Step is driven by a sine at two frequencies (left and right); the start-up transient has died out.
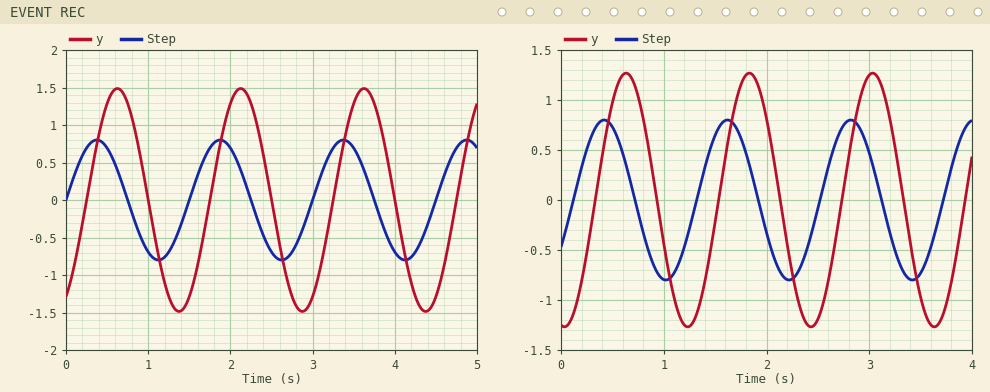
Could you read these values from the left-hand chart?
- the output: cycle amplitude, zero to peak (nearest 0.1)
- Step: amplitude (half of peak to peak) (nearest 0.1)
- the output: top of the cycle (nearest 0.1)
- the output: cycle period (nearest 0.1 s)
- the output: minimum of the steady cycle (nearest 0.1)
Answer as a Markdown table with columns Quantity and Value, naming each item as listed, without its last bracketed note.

| Quantity | Value |
|---|---|
| the output: cycle amplitude, zero to peak | 1.5 |
| Step: amplitude (half of peak to peak) | 0.8 |
| the output: top of the cycle | 1.5 |
| the output: cycle period | 1.5 s |
| the output: minimum of the steady cycle | -1.5 |
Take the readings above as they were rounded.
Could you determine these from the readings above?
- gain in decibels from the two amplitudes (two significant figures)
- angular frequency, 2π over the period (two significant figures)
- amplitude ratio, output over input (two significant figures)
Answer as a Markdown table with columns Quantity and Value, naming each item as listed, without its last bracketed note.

| Quantity | Value |
|---|---|
| gain in decibels from the two amplitudes | 5.5 dB |
| angular frequency, 2π over the period | 4.2 rad/s |
| amplitude ratio, output over input | 1.9 |
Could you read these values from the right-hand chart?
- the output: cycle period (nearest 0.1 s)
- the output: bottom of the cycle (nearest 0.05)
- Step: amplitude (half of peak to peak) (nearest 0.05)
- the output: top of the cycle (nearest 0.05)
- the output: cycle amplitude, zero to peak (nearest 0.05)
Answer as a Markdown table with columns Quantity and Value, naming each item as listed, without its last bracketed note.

| Quantity | Value |
|---|---|
| the output: cycle period | 1.2 s |
| the output: bottom of the cycle | -1.25 |
| Step: amplitude (half of peak to peak) | 0.80 |
| the output: top of the cycle | 1.25 |
| the output: cycle amplitude, zero to peak | 1.25 |
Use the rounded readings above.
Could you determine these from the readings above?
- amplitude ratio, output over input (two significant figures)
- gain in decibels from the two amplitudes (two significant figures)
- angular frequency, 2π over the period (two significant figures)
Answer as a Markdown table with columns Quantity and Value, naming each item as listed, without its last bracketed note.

| Quantity | Value |
|---|---|
| amplitude ratio, output over input | 1.6 |
| gain in decibels from the two amplitudes | 3.9 dB |
| angular frequency, 2π over the period | 5.2 rad/s |
